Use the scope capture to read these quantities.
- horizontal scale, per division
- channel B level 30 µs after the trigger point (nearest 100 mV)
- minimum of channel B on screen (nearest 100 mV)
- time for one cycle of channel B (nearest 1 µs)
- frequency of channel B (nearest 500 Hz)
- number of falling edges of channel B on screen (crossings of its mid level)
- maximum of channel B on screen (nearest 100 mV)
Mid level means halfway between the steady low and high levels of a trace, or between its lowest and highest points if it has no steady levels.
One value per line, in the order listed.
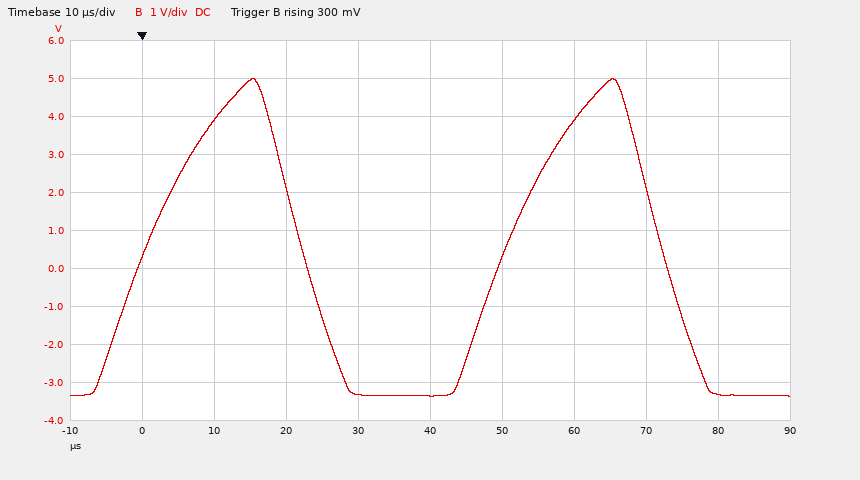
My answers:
10 µs
-3.3 V
-3.4 V
50 µs
20.0 kHz
2
5.0 V
